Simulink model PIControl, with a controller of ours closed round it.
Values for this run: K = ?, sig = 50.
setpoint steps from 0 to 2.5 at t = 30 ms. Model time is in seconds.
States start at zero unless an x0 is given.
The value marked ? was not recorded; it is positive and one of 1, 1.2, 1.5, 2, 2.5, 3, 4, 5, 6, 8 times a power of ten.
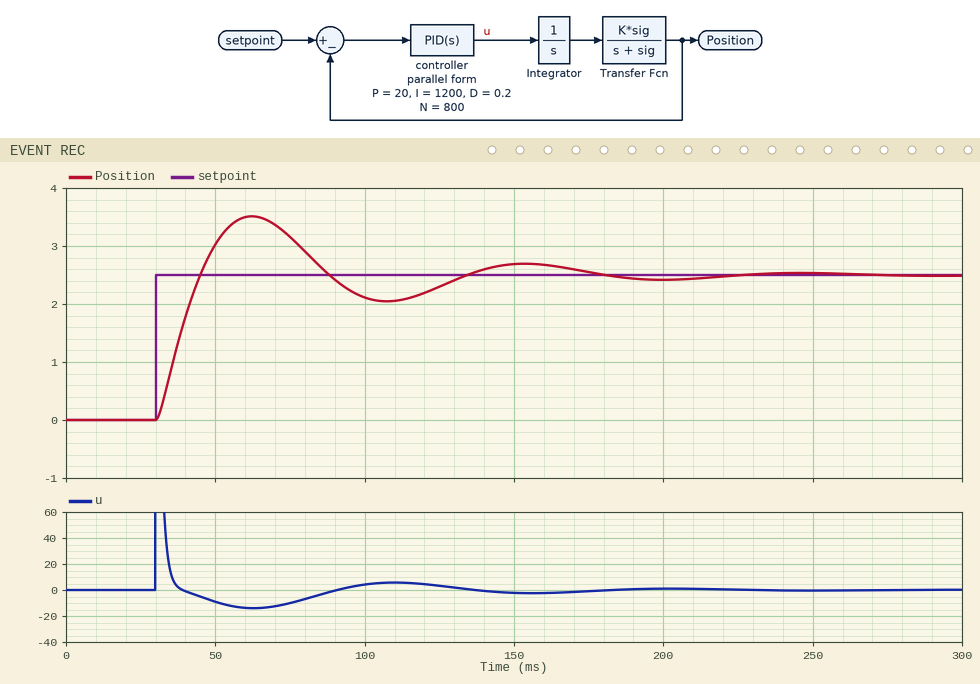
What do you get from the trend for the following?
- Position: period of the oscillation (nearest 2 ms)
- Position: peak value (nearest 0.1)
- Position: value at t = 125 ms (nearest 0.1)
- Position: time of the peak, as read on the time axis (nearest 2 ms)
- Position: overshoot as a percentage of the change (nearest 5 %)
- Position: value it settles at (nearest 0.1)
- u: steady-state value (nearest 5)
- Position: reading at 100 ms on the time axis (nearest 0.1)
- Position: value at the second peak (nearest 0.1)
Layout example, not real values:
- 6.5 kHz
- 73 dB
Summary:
- 92 ms
- 3.5
- 2.3
- 62 ms
- 40 %
- 2.5
- 0
- 2.1
- 2.7
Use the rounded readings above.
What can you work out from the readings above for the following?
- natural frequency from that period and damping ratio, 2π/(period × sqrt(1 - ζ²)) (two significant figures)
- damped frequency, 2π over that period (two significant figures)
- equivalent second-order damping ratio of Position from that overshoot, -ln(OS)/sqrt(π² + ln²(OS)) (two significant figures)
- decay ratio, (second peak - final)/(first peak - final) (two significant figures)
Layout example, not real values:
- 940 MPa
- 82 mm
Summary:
- 0.071 rad/ms
- 0.068 rad/ms
- 0.28
- 0.20
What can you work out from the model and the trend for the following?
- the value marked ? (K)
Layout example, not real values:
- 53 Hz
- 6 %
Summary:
- 8
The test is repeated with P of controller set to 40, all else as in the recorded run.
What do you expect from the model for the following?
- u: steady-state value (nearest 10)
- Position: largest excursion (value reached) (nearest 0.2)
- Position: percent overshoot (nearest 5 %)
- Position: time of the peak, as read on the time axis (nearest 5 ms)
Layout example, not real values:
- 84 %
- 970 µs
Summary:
- 0
- 3.4
- 35 %
- 50 ms
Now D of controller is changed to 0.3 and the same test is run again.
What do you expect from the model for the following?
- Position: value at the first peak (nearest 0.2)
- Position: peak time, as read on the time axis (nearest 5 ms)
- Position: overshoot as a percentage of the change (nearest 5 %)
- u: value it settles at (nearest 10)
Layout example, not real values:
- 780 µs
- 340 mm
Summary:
- 3.2
- 65 ms
- 25 %
- 0
